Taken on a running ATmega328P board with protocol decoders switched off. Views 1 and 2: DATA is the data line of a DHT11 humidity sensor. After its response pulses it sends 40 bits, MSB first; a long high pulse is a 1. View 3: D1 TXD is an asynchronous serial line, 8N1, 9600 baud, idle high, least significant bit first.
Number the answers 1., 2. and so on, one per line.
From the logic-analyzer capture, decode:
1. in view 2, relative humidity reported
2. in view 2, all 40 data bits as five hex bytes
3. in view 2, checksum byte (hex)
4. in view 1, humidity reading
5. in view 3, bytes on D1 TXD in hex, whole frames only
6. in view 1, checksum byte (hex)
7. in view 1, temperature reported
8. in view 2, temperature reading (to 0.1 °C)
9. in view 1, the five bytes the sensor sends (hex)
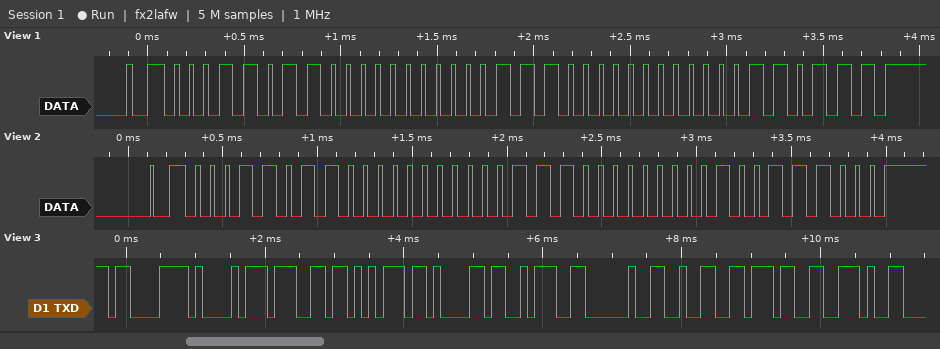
1. 27 %
2. 1B 00 1C 01 38
3. 0x38
4. 27 %
5. C3 A1 67 75 61 3A 20 32 37 2E
6. 0x37
7. 28.0 °C
8. 28.1 °C
9. 1B 00 1C 00 37
